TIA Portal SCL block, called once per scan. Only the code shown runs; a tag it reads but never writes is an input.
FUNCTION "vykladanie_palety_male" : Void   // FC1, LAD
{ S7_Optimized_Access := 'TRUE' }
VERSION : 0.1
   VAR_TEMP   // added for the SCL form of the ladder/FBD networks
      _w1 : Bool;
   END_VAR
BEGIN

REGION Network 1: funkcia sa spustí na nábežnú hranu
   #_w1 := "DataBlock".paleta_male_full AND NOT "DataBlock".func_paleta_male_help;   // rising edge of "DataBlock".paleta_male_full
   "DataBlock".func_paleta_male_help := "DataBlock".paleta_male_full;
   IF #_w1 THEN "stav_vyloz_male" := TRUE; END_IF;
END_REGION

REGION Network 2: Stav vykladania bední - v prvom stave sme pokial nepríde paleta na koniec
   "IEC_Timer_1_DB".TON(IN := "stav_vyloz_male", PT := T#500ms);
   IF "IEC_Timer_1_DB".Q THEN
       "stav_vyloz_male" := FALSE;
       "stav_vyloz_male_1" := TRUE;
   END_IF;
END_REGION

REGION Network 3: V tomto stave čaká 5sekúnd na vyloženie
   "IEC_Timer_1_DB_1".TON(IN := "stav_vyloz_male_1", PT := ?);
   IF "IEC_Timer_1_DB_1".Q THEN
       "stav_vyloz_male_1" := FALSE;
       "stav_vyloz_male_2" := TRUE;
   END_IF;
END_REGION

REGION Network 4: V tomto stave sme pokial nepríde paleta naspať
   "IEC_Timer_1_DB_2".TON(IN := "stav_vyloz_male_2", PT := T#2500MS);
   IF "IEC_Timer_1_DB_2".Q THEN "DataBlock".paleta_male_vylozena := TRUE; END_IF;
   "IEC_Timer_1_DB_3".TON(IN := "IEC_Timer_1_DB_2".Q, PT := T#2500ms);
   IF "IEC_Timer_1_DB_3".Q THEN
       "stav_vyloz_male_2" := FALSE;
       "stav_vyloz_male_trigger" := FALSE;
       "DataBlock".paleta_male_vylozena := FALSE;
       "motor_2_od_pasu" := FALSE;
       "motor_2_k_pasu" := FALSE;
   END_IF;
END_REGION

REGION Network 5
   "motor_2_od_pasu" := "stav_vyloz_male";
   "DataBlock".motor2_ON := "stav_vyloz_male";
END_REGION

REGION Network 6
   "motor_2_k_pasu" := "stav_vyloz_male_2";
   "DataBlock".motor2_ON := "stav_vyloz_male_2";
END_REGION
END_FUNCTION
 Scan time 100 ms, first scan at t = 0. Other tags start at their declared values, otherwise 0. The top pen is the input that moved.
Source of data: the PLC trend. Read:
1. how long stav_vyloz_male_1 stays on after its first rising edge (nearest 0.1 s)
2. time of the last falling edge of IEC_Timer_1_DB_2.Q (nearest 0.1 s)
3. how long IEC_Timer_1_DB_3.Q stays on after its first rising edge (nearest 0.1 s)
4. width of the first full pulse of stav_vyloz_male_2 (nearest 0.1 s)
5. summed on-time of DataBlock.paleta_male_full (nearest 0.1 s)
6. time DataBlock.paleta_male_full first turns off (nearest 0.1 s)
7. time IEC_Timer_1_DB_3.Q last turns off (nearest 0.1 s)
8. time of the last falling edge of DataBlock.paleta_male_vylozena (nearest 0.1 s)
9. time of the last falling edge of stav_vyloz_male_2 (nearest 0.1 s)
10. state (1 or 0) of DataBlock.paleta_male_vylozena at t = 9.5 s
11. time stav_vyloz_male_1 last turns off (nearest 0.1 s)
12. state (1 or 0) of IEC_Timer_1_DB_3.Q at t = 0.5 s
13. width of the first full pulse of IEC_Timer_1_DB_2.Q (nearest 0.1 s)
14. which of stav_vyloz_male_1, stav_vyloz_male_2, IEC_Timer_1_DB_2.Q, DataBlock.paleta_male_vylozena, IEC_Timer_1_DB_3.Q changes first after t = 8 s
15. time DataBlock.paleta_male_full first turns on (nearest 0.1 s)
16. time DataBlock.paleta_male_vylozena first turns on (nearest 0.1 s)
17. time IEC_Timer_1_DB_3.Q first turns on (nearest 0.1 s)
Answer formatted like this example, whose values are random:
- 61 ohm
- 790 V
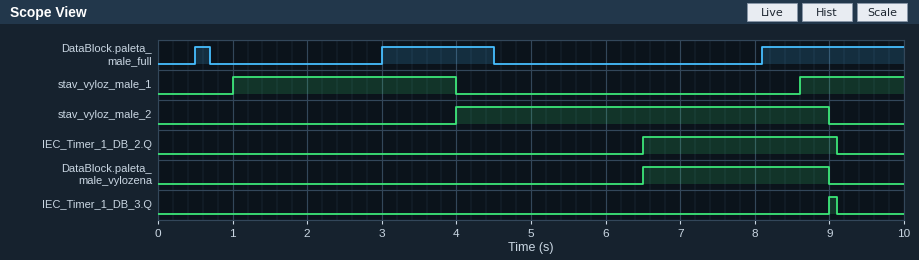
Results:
- 3.0 s
- 9.1 s
- 0.1 s
- 5.0 s
- 3.6 s
- 0.7 s
- 9.1 s
- 9.0 s
- 9.0 s
- 0
- 4.0 s
- 0
- 2.6 s
- stav_vyloz_male_1
- 0.5 s
- 6.5 s
- 9.0 s
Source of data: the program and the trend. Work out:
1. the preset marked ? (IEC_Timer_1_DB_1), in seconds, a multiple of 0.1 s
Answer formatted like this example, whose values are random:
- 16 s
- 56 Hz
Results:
- 3.0 s
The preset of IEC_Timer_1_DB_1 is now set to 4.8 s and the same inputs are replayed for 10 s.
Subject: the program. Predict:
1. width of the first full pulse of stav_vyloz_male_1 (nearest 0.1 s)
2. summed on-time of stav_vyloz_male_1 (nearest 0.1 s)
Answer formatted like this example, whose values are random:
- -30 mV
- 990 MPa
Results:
- 4.8 s
- 6.2 s
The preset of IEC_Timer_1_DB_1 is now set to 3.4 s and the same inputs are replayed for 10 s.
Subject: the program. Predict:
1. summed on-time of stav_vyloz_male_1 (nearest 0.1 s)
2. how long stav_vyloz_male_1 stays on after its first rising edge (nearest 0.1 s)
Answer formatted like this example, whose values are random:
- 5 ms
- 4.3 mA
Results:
- 4.8 s
- 3.4 s
